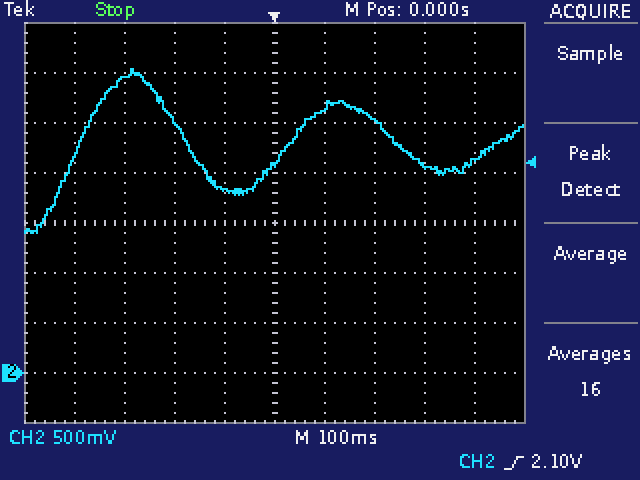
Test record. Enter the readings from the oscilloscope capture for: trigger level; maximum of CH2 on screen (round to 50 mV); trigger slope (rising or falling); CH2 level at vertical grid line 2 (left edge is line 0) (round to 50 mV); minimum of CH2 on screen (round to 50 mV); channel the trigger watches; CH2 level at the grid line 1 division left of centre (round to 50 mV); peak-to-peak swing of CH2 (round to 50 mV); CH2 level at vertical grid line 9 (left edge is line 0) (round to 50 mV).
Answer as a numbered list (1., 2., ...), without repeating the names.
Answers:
1. 2.10 V
2. 3.05 V
3. rising
4. 2.95 V
5. 1.40 V
6. CH2
7. 1.85 V
8. 1.65 V
9. 2.10 V
